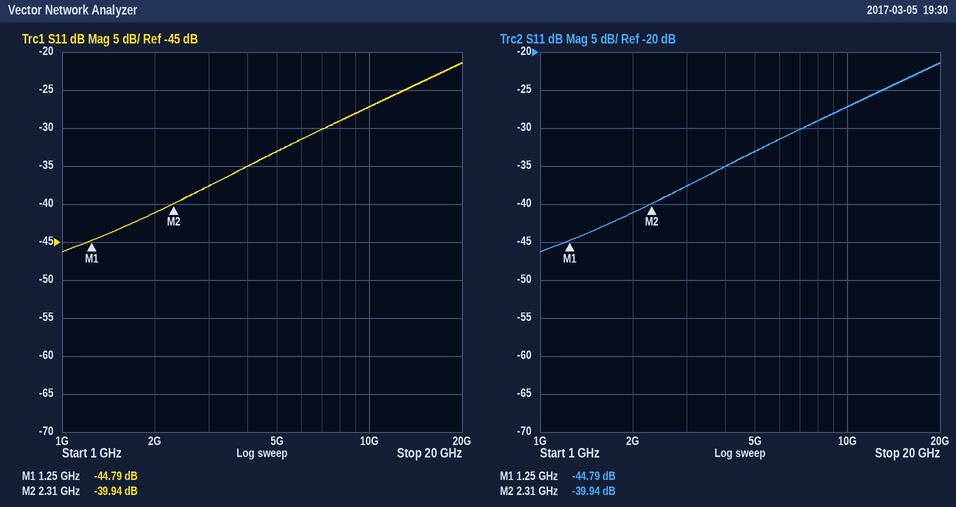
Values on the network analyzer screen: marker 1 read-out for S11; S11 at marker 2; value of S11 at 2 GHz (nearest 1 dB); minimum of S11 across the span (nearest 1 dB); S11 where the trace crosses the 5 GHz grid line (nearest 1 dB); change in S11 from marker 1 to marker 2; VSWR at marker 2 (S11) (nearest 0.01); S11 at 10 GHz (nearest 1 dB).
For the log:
-44.79 dB
-39.94 dB
-41 dB
-46 dB
-33 dB
4.85 dB
1.02
-27 dB
